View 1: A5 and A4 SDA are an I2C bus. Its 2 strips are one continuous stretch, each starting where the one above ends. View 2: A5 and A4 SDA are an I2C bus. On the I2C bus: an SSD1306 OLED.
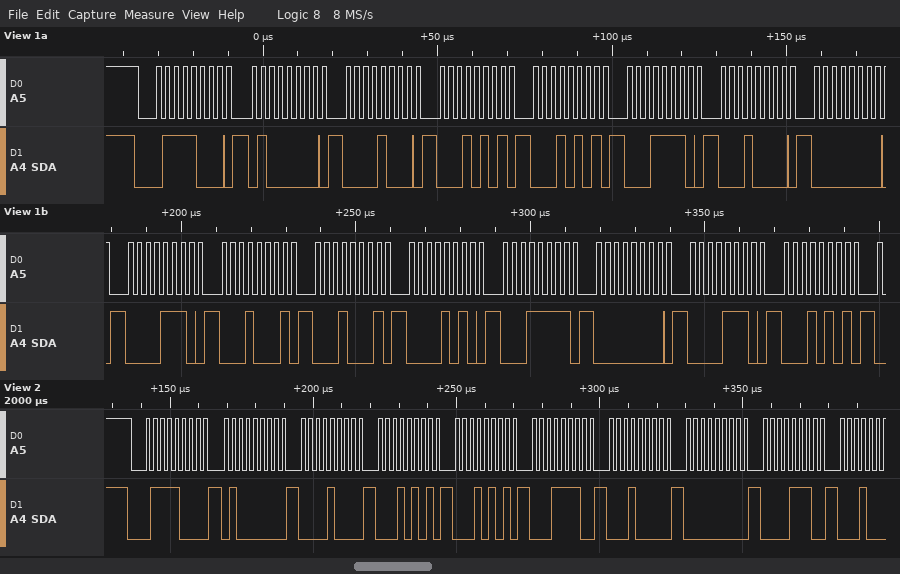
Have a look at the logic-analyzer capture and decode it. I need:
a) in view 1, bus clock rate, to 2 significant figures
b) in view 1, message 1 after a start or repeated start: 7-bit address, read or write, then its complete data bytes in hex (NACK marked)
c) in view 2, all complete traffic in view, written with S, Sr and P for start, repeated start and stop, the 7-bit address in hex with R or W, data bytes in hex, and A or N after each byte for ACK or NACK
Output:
400 kHz
0x3C write: 40 08 15 15 1E 10 00 0E 11 11 0A 1F 00 0E 15
S 3CW A 40 A 08 A 15 A 15 A 1E A 10 A 00 A 0E A
